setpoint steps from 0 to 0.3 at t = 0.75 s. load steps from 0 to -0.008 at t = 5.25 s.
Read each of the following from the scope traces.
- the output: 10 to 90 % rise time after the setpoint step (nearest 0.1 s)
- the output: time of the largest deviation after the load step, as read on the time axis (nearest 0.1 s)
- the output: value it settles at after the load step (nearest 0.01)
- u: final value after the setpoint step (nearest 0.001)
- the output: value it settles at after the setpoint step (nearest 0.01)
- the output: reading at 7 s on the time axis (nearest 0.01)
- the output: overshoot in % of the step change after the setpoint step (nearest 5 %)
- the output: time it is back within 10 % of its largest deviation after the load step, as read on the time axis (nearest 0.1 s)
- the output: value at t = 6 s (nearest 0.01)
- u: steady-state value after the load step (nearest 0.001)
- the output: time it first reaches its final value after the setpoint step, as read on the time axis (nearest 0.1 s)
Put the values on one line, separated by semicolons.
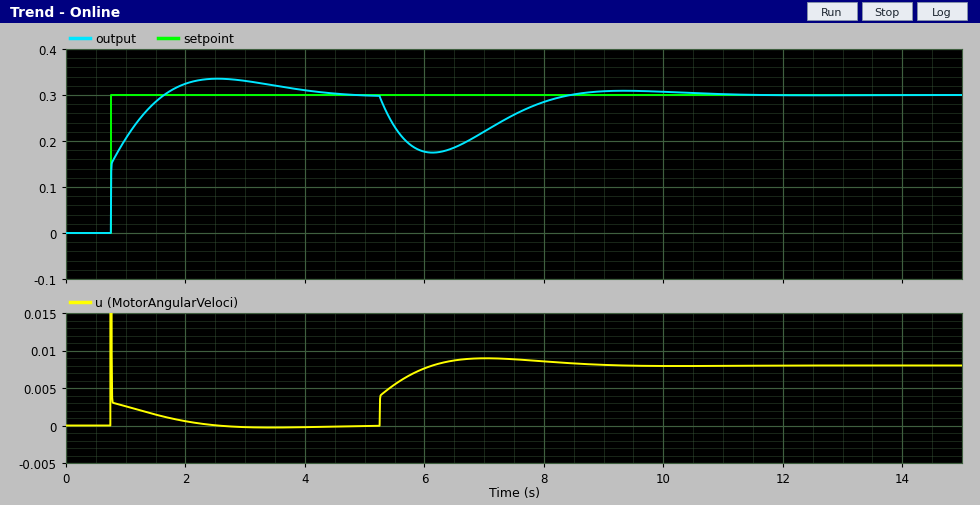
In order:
0.6 s; 6.1 s; 0.30; 0.000; 0.30; 0.22; 10 %; 8.1 s; 0.18; 0.008; 1.6 s
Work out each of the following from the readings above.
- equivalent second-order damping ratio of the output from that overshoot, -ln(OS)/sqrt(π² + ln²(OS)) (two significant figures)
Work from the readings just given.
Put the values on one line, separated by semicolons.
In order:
0.59
